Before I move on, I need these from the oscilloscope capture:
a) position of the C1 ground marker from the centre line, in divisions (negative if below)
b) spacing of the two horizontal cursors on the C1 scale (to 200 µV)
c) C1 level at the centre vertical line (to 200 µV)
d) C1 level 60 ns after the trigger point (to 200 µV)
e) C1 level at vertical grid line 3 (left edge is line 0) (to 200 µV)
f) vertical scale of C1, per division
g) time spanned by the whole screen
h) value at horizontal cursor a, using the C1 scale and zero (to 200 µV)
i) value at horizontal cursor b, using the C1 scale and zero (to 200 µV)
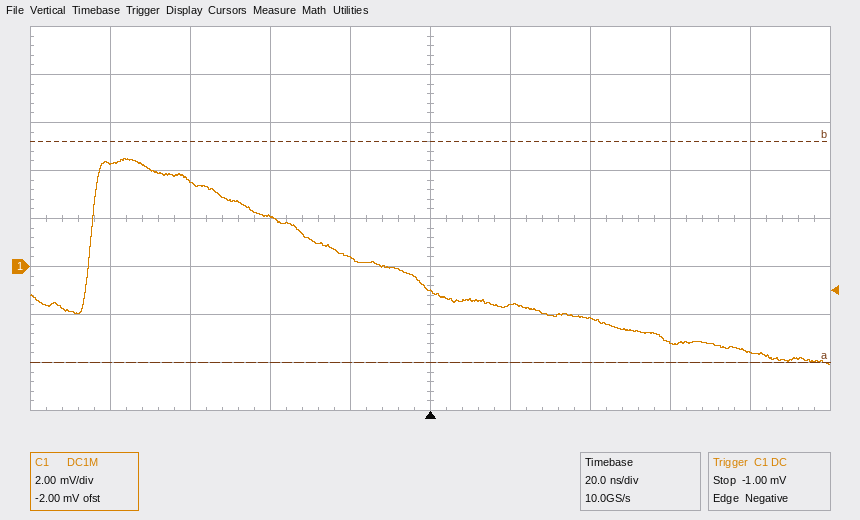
-1.0 div
9.2 mV
-1.0 mV
-3.2 mV
2.0 mV
2 mV
200 ns
-4.0 mV
5.2 mV
